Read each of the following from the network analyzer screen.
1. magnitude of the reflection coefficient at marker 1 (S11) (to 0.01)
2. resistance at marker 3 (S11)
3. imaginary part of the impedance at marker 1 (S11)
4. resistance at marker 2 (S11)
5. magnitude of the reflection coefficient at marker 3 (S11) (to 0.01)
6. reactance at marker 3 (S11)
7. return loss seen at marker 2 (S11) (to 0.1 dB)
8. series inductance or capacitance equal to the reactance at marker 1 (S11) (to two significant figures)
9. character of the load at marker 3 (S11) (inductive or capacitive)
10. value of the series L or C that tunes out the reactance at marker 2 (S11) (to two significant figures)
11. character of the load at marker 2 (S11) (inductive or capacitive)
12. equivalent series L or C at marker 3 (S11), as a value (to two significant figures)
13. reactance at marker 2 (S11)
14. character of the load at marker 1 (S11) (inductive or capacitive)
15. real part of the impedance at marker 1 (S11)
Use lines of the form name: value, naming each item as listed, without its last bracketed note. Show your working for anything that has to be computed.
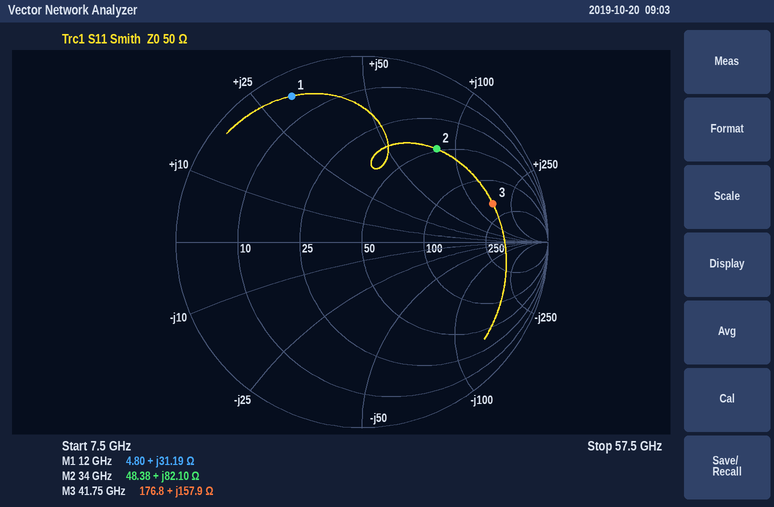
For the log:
magnitude of the reflection coefficient at marker 1 (S11): 0.87
resistance at marker 3: 176.8 Ω
imaginary part of the impedance at marker 1: +31.19 Ω
resistance at marker 2: 48.38 Ω
magnitude of the reflection coefficient at marker 3 (S11): 0.73
reactance at marker 3: +157.9 Ω
return loss seen at marker 2 (S11): 3.9 dB
series inductance or capacitance equal to the reactance at marker 1 (S11): L = 31.19 Ω/(2π × 12 GHz) ≈ 414 pH, so 410 pH to two significant figures
character of the load at marker 3 (S11): inductive
value of the series L or C that tunes out the reactance at marker 2 (S11): C = 1/(2π × 34 GHz × 82.1 Ω) ≈ 57 fF
character of the load at marker 2 (S11): inductive
equivalent series L or C at marker 3 (S11), as a value: L = 157.9 Ω/(2π × 41.75 GHz) ≈ 602 pH, so 600 pH to two significant figures
reactance at marker 2: +82.10 Ω
character of the load at marker 1 (S11): inductive
real part of the impedance at marker 1: 4.80 Ω
